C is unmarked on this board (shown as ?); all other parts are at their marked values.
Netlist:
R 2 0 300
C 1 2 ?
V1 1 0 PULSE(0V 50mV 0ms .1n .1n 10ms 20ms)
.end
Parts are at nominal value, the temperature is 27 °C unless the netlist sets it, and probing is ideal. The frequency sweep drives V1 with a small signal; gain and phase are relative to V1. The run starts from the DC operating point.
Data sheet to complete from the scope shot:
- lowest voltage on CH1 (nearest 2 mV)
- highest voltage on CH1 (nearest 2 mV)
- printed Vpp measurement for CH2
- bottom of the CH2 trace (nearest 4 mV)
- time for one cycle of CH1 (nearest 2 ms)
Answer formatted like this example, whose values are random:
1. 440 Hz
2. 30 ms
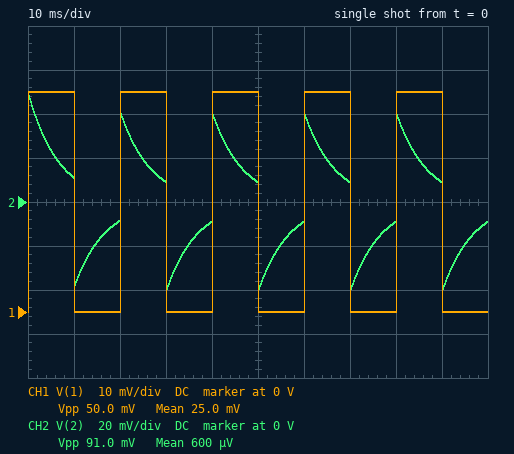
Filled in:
1. 0 V
2. 50 mV
3. 91.0 mV
4. -40 mV
5. 20 ms
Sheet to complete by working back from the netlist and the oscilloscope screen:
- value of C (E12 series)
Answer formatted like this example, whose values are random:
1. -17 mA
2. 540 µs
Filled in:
1. 22 µF
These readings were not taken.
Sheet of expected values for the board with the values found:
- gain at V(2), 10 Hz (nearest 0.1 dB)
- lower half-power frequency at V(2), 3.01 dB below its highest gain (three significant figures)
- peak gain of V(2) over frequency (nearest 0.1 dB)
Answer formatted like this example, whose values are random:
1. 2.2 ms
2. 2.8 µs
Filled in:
1. -8.3 dB
2. 24.1 Hz
3. 0 dB
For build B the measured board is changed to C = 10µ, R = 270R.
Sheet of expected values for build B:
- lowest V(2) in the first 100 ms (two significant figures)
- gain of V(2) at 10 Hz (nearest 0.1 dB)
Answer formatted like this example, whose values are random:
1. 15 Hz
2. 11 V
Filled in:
1. -49 mV
2. -15.5 dB
